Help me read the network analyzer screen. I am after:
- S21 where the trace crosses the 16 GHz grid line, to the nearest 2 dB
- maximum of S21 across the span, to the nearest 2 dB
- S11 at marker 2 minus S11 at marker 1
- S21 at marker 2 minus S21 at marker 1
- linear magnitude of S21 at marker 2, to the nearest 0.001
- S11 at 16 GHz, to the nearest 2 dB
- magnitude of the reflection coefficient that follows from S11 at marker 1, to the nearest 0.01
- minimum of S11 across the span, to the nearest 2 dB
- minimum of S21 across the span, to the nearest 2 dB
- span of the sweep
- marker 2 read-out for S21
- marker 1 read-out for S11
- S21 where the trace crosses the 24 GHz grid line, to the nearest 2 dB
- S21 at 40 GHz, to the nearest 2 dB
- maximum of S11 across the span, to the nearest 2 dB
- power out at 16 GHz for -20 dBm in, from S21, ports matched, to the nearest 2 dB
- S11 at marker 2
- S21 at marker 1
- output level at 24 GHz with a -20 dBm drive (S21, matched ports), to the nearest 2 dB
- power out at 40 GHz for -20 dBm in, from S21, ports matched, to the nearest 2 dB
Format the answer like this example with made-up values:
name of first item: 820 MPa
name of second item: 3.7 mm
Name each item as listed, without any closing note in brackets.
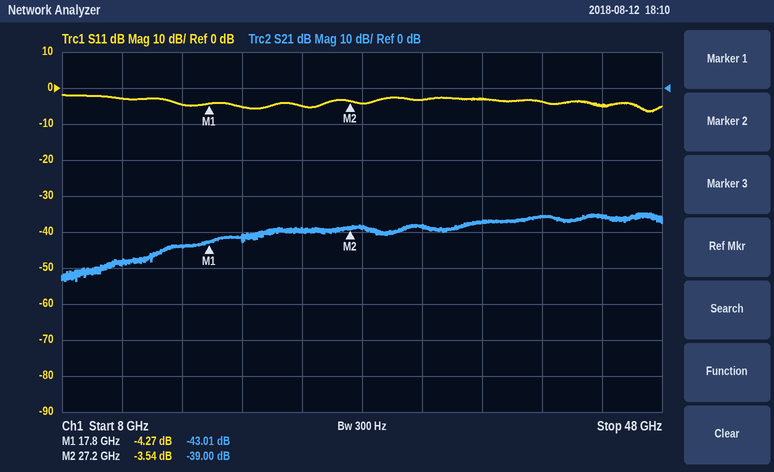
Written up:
S21 where the trace crosses the 16 GHz grid line, to the nearest 2 dB: -44 dB
maximum of S21 across the span, to the nearest 2 dB: -34 dB
S11 at marker 2 minus S11 at marker 1: 0.73 dB
S21 at marker 2 minus S21 at marker 1: 4.01 dB
linear magnitude of S21 at marker 2, to the nearest 0.001: 0.011
S11 at 16 GHz, to the nearest 2 dB: -4 dB
magnitude of the reflection coefficient that follows from S11 at marker 1, to the nearest 0.01: 0.61
minimum of S11 across the span, to the nearest 2 dB: -6 dB
minimum of S21 across the span, to the nearest 2 dB: -54 dB
span of the sweep: 40 GHz
marker 2 read-out for S21: -39.00 dB
marker 1 read-out for S11: -4.27 dB
S21 where the trace crosses the 24 GHz grid line, to the nearest 2 dB: -40 dB
S21 at 40 GHz, to the nearest 2 dB: -36 dB
maximum of S11 across the span, to the nearest 2 dB: -2 dB
power out at 16 GHz for -20 dBm in, from S21, ports matched, to the nearest 2 dB: -64 dBm
S11 at marker 2: -3.54 dB
S21 at marker 1: -43.01 dB
output level at 24 GHz with a -20 dBm drive (S21, matched ports), to the nearest 2 dB: -60 dBm
power out at 40 GHz for -20 dBm in, from S21, ports matched, to the nearest 2 dB: -56 dBm
